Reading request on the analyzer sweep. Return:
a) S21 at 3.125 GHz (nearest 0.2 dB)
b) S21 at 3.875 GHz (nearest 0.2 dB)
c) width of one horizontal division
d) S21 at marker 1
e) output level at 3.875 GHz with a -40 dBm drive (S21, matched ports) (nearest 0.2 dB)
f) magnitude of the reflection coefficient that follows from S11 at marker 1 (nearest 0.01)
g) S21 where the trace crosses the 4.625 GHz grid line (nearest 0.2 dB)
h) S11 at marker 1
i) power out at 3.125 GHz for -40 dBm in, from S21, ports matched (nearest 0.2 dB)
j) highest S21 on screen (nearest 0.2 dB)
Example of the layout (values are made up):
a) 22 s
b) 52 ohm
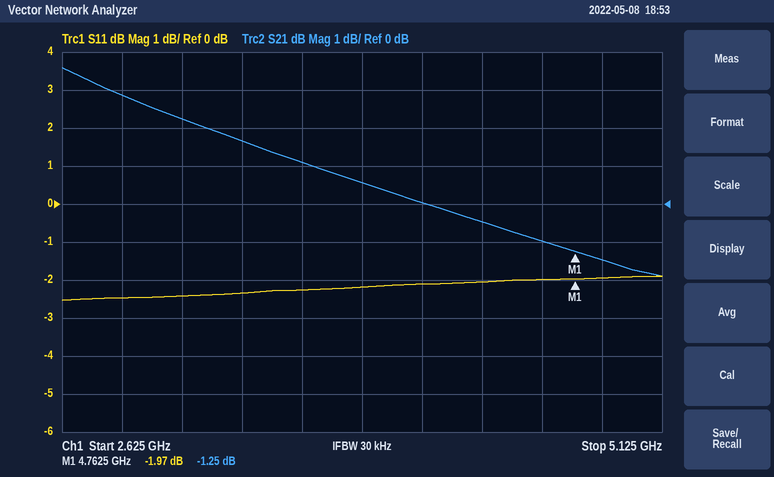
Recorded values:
a) 2.2 dB
b) 0.6 dB
c) 250 MHz
d) -1.25 dB
e) -39.4 dBm
f) 0.80
g) -1.0 dB
h) -1.97 dB
i) -37.8 dBm
j) 3.6 dB
